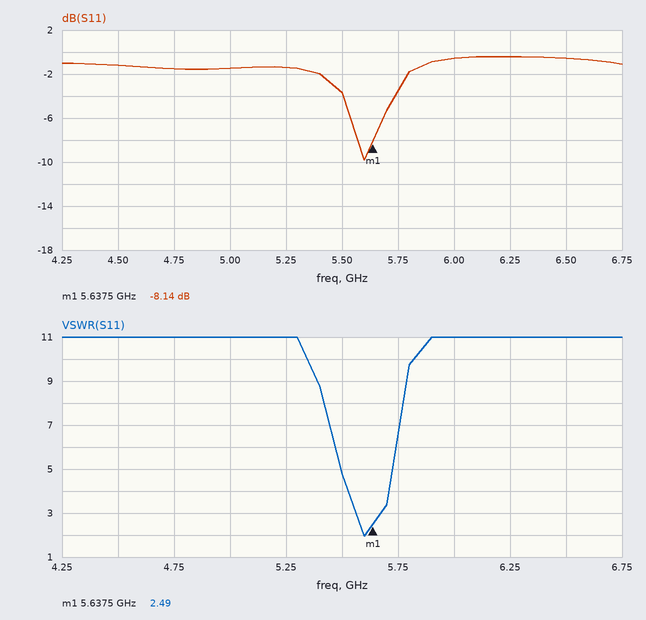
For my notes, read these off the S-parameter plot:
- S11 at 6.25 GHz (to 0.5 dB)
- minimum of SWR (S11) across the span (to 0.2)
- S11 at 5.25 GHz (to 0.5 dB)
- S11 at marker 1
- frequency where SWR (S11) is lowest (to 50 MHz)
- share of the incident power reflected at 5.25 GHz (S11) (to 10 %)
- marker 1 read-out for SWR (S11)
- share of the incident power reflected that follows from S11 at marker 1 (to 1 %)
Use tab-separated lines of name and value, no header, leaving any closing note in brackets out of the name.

S11 at 6.25 GHz	-0.5 dB
minimum of SWR (S11) across the span	2.0
S11 at 5.25 GHz	-1.5 dB
S11 at marker 1	-8.14 dB
frequency where SWR (S11) is lowest	5.60 GHz
share of the incident power reflected at 5.25 GHz (S11)	70 %
marker 1 read-out for SWR	2.49
share of the incident power reflected that follows from S11 at marker 1	15 %
